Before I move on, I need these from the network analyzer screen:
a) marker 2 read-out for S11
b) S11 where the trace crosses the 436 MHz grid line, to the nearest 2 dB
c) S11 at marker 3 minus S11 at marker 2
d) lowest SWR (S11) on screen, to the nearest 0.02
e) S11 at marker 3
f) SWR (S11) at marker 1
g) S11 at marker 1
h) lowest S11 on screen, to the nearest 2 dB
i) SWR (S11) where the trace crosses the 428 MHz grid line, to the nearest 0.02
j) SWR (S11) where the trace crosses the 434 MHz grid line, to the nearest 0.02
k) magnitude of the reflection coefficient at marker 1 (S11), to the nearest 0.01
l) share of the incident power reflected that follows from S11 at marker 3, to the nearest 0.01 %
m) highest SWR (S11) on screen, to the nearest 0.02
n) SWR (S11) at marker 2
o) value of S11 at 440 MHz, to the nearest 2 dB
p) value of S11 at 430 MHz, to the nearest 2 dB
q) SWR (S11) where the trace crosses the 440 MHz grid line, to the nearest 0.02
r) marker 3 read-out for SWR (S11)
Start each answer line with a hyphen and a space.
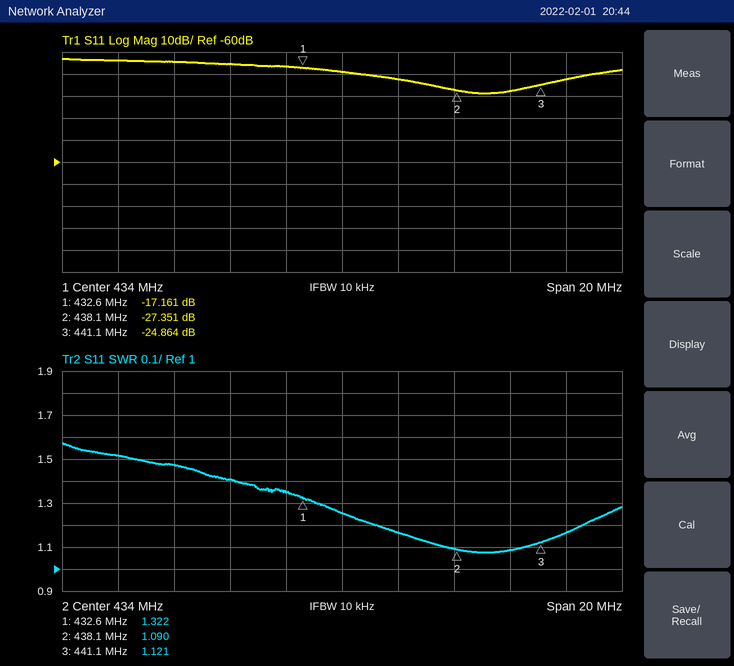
- -27.351 dB
- -22 dB
- 2.487 dB
- 1.08
- -24.864 dB
- 1.322
- -17.161 dB
- -28 dB
- 1.48
- 1.26
- 0.14
- 0.33 %
- 1.58
- 1.090
- -28 dB
- -16 dB
- 1.08
- 1.121
